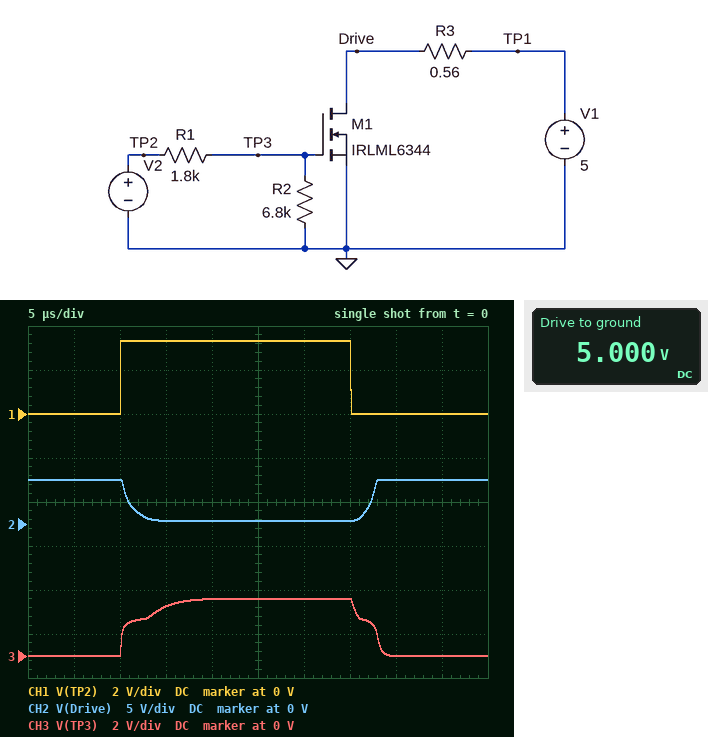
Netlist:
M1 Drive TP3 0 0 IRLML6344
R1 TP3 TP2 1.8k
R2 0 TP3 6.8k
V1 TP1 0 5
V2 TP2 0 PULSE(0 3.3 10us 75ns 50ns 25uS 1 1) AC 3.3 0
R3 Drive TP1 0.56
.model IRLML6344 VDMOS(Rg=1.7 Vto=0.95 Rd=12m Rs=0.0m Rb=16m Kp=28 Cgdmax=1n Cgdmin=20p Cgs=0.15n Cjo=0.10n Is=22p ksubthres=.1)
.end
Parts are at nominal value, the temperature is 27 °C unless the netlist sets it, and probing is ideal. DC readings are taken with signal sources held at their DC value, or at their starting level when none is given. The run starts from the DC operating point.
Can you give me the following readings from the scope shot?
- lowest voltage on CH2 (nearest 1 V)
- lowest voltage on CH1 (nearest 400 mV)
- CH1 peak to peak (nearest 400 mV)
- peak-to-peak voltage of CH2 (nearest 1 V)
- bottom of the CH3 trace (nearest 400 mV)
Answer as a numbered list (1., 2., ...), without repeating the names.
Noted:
1. 0 V
2. 0 V
3. 3.2 V
4. 5 V
5. 0 V
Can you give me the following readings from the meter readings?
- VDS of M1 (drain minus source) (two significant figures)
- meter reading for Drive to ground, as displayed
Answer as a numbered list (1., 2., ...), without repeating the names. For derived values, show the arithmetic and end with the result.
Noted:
1. 5 V = 5.0 V
2. 5.000 V
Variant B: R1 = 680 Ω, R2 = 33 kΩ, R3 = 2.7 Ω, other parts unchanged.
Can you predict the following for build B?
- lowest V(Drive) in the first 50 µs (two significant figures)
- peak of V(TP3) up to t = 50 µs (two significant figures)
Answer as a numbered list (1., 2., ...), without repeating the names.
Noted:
1. 51 mV
2. 3.2 V
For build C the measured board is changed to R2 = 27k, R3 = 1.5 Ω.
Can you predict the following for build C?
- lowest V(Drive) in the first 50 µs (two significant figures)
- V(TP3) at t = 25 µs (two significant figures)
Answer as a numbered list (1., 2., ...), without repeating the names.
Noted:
1. 94 mV
2. 3.1 V
